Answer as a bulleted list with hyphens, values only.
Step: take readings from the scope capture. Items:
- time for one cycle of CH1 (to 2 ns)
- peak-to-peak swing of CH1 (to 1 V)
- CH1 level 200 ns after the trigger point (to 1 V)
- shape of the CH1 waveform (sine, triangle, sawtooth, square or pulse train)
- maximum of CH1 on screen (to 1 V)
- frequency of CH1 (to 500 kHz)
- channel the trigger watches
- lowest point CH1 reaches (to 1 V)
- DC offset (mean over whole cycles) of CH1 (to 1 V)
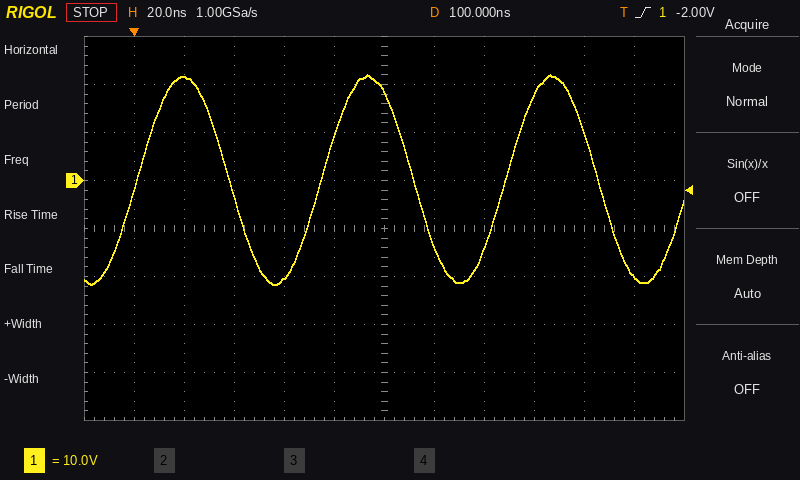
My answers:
- 74 ns
- 44 V
- -20 V
- sine
- 22 V
- 13.5 MHz
- CH1
- -22 V
- 0 V
